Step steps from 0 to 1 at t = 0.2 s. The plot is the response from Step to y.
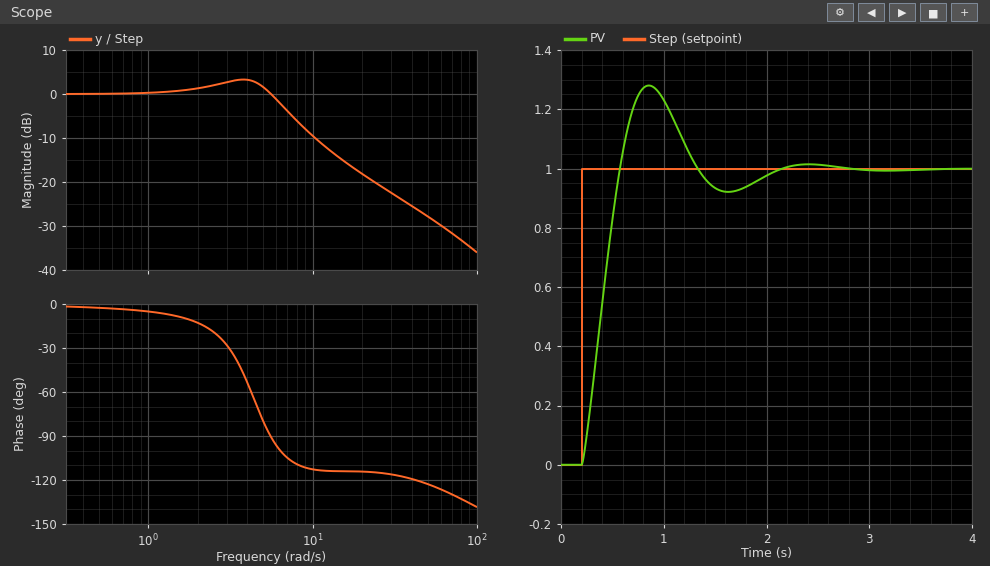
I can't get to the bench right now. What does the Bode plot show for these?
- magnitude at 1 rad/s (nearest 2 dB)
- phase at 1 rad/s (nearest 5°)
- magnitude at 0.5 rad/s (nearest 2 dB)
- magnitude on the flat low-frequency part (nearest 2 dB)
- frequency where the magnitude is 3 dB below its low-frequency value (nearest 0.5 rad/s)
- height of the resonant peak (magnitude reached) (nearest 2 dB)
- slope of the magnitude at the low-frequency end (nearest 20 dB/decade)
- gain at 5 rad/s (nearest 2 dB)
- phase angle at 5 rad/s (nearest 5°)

0 dB
-5°
0 dB
0 dB
6.5 rad/s
4 dB
0 dB/decade
2 dB
-80°
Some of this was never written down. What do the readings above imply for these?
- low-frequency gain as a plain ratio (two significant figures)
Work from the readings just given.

1.0
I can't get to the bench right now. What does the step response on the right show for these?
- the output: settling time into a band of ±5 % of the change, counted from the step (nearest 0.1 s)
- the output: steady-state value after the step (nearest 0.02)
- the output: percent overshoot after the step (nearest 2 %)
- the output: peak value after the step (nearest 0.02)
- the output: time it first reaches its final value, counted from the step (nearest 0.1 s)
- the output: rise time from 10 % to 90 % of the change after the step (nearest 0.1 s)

1.7 s
1.00
28 %
1.28
0.4 s
0.3 s
